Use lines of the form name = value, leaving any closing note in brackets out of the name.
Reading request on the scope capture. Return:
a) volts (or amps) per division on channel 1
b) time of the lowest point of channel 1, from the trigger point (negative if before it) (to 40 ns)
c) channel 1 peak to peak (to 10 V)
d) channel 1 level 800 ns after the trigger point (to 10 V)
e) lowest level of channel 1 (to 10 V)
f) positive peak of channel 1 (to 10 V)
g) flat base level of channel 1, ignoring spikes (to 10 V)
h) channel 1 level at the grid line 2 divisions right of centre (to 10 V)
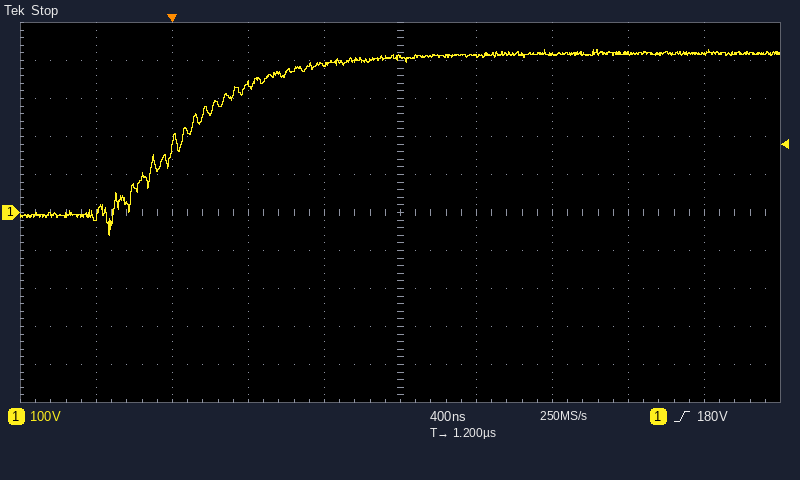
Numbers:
volts (or amps) per division on channel 1 = 100 V
time of the lowest point of channel 1, from the trigger point (negative if before it) = -320 ns
channel 1 peak to peak = 490 V
channel 1 level 800 ns after the trigger point = 390 V
lowest level of channel 1 = -60 V
positive peak of channel 1 = 430 V
flat base level of channel 1, ignoring spikes = -10 V
channel 1 level at the grid line 2 divisions right of centre = 420 V
